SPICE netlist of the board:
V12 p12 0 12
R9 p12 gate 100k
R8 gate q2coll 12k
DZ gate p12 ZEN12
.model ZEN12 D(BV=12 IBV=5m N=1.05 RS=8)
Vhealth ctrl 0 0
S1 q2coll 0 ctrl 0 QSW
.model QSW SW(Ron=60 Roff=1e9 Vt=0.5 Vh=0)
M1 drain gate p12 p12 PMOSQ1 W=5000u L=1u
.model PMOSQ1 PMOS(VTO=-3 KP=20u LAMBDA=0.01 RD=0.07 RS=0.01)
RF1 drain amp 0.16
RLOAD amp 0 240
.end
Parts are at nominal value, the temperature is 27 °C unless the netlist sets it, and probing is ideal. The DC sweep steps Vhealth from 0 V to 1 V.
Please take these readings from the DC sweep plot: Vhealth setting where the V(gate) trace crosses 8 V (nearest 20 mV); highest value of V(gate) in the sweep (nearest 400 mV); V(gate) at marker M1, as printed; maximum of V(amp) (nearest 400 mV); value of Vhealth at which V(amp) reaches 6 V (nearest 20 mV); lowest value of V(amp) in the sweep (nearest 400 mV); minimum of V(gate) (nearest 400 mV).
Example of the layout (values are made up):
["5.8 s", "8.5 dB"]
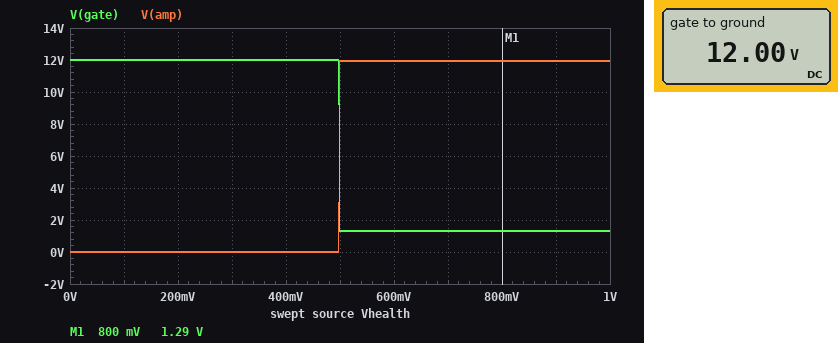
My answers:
["500 mV", "12.0 V", "1.29 V", "12.0 V", "500 mV", "0 V", "1.2 V"]
